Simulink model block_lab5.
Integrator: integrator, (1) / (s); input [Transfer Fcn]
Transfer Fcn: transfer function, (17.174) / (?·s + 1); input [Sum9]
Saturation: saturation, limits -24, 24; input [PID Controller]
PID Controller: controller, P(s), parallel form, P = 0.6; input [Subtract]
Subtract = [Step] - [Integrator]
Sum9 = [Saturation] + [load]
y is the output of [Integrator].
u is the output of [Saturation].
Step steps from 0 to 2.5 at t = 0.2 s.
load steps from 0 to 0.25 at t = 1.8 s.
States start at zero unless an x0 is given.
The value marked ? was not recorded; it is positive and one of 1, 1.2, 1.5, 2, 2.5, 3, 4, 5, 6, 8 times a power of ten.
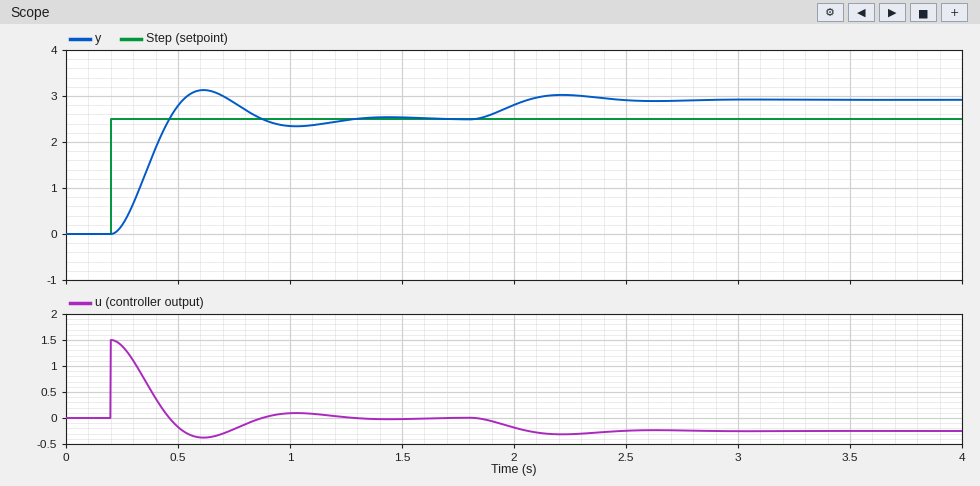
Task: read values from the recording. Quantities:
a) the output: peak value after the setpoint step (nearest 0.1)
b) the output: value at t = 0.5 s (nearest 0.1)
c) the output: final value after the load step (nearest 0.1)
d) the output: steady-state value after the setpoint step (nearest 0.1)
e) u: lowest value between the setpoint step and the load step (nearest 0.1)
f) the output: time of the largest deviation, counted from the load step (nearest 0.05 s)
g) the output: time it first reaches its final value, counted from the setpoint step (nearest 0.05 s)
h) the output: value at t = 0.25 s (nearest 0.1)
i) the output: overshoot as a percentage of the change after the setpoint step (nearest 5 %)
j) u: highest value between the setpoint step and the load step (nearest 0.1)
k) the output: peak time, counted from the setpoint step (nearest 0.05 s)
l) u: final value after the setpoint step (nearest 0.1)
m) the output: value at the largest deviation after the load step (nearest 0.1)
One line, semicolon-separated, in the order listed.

3.1; 2.8; 2.9; 2.5; -0.4; 0.40 s; 0.25 s; 0.2; 25 %; 1.5; 0.40 s; 0.0; 3.0
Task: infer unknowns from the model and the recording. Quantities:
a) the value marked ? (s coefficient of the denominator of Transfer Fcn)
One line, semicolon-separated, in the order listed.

0.15
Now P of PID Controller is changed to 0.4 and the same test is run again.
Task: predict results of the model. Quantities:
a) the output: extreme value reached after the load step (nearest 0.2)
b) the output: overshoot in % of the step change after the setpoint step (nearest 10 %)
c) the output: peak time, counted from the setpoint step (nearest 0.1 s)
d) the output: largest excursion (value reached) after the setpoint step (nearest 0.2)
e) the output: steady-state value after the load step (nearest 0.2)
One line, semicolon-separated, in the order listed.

3.2; 20 %; 0.5 s; 3.0; 3.2
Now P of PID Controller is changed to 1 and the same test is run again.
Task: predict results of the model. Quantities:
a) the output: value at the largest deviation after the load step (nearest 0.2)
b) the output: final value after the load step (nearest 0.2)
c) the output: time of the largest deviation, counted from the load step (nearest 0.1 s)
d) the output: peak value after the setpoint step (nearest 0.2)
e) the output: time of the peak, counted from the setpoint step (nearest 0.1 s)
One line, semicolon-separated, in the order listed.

2.8; 2.8; 0.3 s; 3.4; 0.3 s
